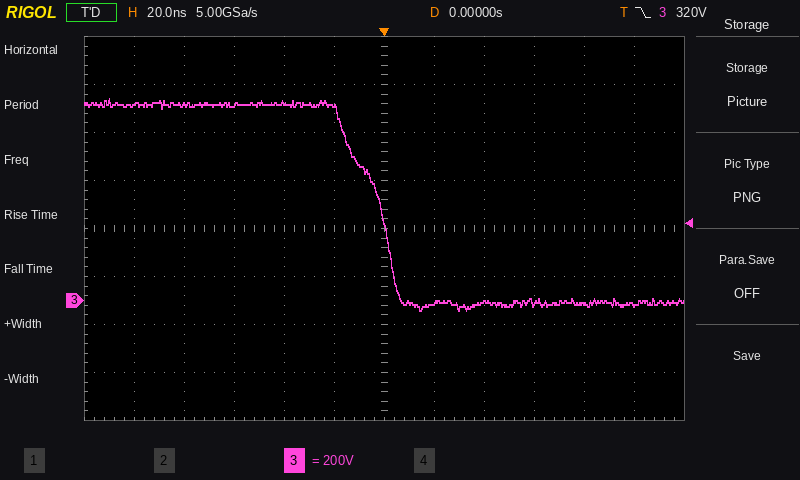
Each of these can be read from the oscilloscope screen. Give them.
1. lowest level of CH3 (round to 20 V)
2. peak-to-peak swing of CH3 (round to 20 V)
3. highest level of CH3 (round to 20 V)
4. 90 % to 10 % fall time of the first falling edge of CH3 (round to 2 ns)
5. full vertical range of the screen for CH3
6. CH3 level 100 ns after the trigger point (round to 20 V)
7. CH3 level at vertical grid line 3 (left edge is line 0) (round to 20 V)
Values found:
-40 V
880 V
840 V
22 ns
1.6 kV
-20 V
820 V
